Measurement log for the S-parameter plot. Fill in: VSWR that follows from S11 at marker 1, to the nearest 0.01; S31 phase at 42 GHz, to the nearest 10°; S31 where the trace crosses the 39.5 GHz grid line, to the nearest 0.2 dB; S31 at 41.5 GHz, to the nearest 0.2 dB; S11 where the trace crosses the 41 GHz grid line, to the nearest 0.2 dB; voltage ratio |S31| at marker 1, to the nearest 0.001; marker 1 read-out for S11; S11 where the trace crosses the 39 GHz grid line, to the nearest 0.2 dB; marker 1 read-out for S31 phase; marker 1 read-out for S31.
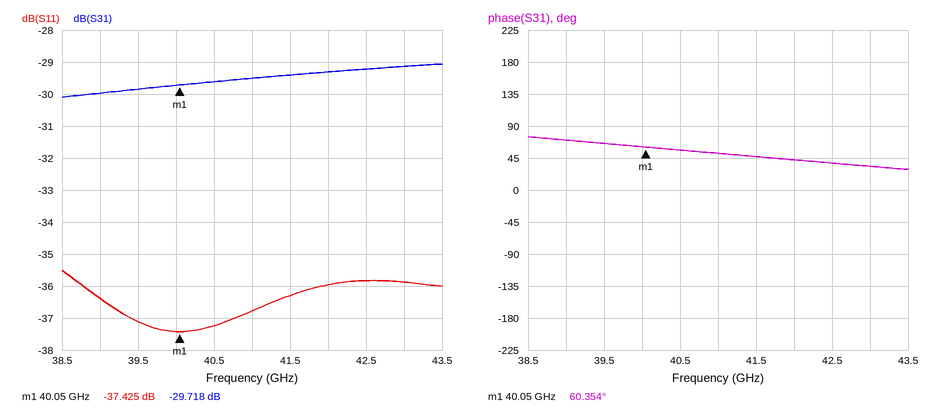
1.03
40°
-29.8 dB
-29.4 dB
-36.8 dB
0.033
-37.425 dB
-36.4 dB
60.354°
-29.718 dB
